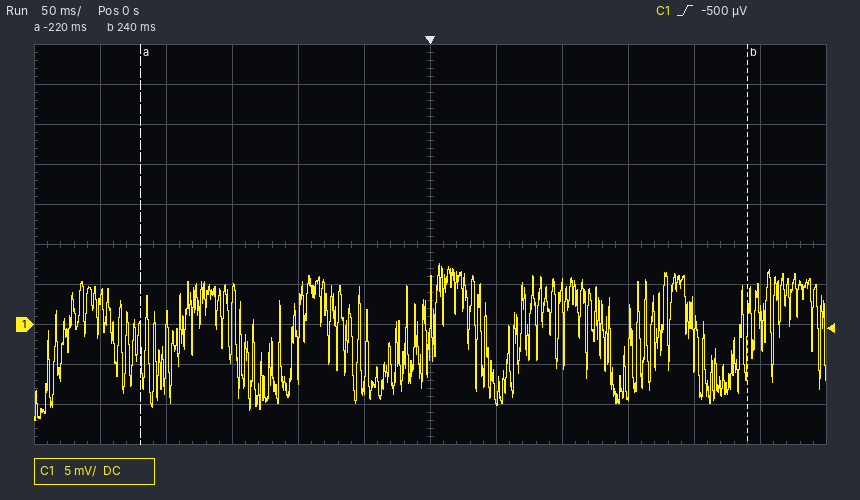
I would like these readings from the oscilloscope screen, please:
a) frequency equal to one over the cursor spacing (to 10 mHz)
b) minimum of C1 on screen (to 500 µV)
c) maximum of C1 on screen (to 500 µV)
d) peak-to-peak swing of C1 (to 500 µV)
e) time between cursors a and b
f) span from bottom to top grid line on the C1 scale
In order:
2.17 Hz
-12.0 mV
7.5 mV
19.5 mV
460 ms
50 mV
